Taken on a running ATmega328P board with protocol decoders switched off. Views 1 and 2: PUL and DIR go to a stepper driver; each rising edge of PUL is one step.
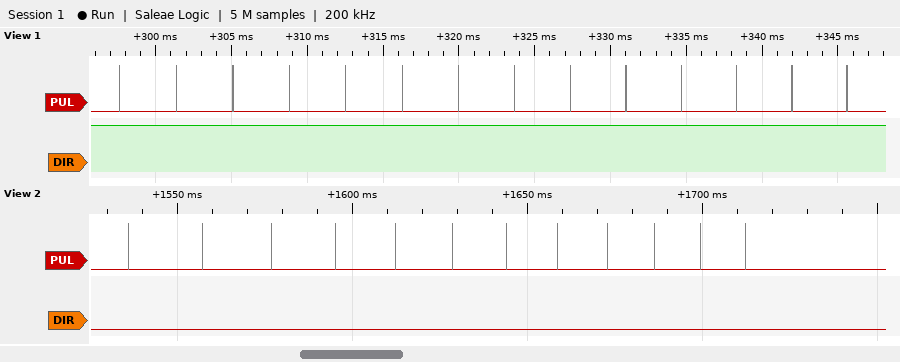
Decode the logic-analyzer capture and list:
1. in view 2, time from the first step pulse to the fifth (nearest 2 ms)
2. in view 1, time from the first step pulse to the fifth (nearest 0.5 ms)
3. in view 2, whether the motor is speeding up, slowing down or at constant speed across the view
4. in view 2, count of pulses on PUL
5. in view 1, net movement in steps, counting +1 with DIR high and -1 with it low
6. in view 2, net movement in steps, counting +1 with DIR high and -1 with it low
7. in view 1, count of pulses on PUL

76 ms
15.0 ms
speeding up
12
+14
-12
14
